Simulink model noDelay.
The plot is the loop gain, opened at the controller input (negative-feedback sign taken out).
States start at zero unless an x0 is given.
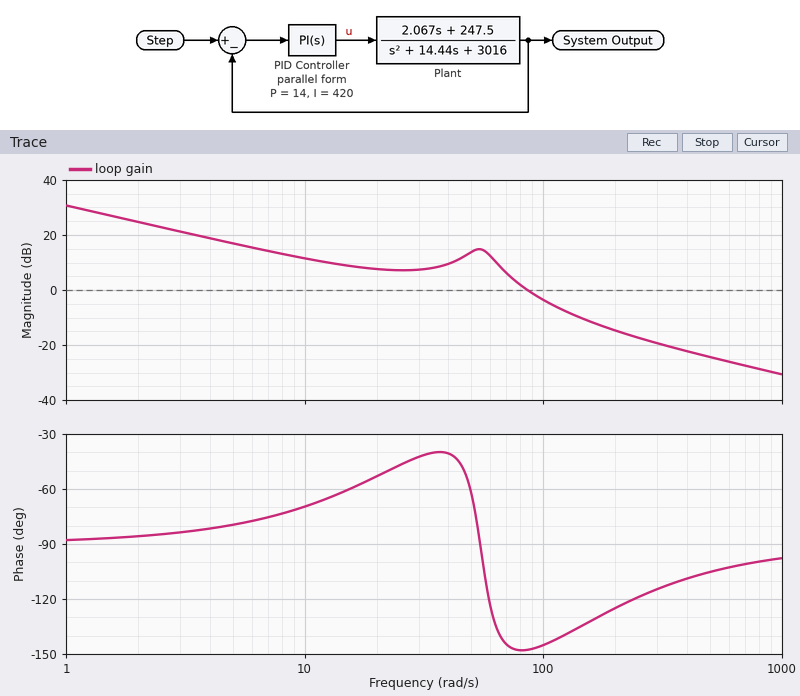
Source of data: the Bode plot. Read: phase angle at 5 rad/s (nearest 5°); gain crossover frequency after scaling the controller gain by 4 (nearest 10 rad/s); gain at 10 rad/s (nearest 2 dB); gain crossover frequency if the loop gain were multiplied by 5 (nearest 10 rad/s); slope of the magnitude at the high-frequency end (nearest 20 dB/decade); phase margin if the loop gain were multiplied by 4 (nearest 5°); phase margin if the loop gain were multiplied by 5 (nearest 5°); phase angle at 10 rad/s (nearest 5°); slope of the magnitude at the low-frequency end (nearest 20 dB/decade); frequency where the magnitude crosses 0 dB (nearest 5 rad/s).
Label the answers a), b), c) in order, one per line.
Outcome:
a) -80°
b) 160 rad/s
c) 12 dB
d) 190 rad/s
e) -20 dB/decade
f) 50°
g) 55°
h) -70°
i) -20 dB/decade
j) 85 rad/s
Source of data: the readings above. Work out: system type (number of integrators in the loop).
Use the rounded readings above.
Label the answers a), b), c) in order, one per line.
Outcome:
a) 1
